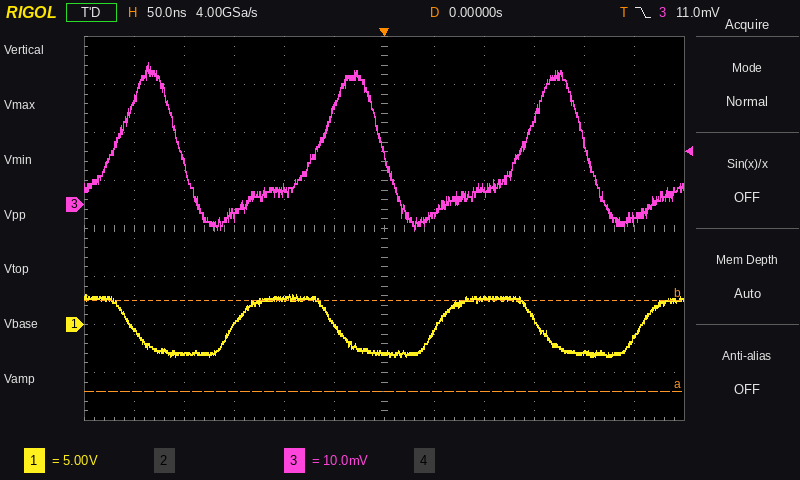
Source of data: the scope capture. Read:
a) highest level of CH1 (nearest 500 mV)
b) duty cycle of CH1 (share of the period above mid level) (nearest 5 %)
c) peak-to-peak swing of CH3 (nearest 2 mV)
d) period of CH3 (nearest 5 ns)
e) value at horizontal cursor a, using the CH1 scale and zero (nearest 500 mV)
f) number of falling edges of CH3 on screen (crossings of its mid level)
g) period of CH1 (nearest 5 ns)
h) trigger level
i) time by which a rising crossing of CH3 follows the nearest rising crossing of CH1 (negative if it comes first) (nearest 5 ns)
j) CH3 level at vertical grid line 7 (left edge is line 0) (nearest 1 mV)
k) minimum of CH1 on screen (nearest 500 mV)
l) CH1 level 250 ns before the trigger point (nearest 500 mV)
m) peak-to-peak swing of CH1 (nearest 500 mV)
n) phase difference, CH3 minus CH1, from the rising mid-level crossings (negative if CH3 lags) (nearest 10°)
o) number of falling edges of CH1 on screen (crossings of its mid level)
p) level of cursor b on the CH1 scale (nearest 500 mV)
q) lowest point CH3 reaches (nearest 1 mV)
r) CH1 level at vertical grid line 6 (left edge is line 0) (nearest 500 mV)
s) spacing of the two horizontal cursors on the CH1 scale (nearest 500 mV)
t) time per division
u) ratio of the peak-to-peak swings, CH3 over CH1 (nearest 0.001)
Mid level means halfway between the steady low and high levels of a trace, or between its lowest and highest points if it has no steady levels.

3.0 V
50 %
34 mV
205 ns
-7.0 V
3
205 ns
11.0 mV
+85 ns
-2 mV
-3.5 V
-500 mV
6.5 V
-150°
3
2.5 V
-5 mV
-3.0 V
9.5 V
50 ns
0.005
